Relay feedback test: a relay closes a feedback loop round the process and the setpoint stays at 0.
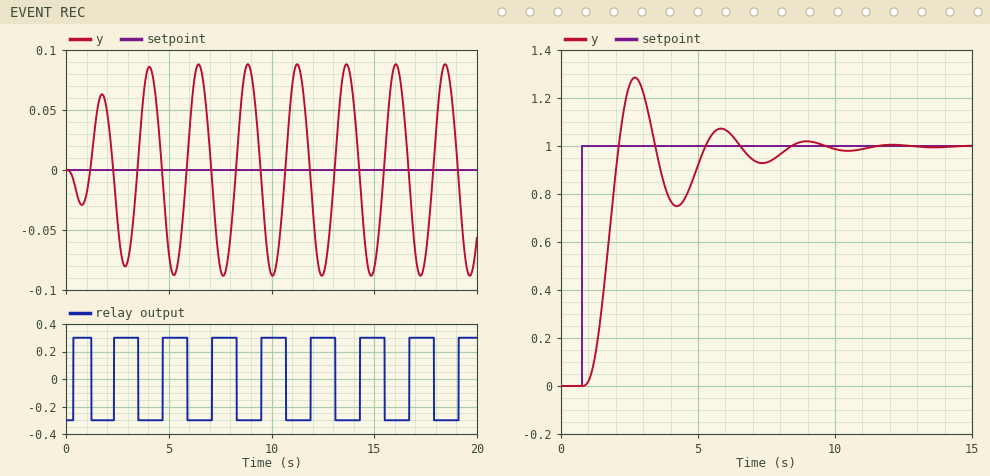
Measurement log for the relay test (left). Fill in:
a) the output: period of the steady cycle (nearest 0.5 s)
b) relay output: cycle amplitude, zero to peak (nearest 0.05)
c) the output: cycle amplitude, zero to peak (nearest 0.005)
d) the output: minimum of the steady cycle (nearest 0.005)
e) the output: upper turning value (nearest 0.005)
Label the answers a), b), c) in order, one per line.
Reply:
a) 2.5 s
b) 0.30
c) 0.090
d) -0.090
e) 0.090
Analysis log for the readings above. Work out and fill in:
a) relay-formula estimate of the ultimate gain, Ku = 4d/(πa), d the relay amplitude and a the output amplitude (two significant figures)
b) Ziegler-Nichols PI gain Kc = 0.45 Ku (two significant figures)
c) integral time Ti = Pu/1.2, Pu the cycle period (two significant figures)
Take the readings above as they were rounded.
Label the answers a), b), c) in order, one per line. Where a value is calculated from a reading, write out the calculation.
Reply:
a) 4 × 0.3 / (π × 0.09) = 4.2
b) 0.45 × 4.2 = 1.9
c) 2.5 / 1.2 = 2.1 s
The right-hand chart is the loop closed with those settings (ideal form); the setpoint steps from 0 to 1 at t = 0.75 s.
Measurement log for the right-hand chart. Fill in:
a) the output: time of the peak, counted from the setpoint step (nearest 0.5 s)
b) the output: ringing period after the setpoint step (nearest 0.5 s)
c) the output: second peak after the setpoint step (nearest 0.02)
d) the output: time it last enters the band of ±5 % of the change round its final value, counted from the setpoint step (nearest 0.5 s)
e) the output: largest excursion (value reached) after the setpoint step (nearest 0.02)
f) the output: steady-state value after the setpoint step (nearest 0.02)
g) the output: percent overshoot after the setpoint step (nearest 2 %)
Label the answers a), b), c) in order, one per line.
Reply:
a) 2.0 s
b) 3.0 s
c) 1.08
d) 7.0 s
e) 1.28
f) 1.00
g) 28 %
